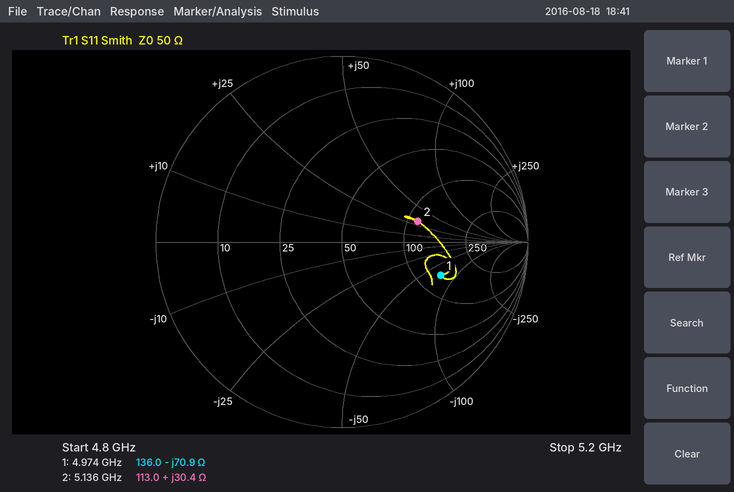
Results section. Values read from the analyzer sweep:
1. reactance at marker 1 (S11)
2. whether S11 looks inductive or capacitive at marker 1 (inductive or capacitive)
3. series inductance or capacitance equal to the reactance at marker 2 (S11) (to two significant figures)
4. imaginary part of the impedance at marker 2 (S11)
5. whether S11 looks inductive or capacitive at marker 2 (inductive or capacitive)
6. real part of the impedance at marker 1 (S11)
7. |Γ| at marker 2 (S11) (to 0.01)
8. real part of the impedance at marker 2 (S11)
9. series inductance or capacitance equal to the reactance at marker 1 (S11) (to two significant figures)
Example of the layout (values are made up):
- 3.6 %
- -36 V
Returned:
- -70.9 Ω
- capacitive
- 940 pH
- +30.4 Ω
- inductive
- 136.0 Ω
- 0.42
- 113.0 Ω
- 450 fF
